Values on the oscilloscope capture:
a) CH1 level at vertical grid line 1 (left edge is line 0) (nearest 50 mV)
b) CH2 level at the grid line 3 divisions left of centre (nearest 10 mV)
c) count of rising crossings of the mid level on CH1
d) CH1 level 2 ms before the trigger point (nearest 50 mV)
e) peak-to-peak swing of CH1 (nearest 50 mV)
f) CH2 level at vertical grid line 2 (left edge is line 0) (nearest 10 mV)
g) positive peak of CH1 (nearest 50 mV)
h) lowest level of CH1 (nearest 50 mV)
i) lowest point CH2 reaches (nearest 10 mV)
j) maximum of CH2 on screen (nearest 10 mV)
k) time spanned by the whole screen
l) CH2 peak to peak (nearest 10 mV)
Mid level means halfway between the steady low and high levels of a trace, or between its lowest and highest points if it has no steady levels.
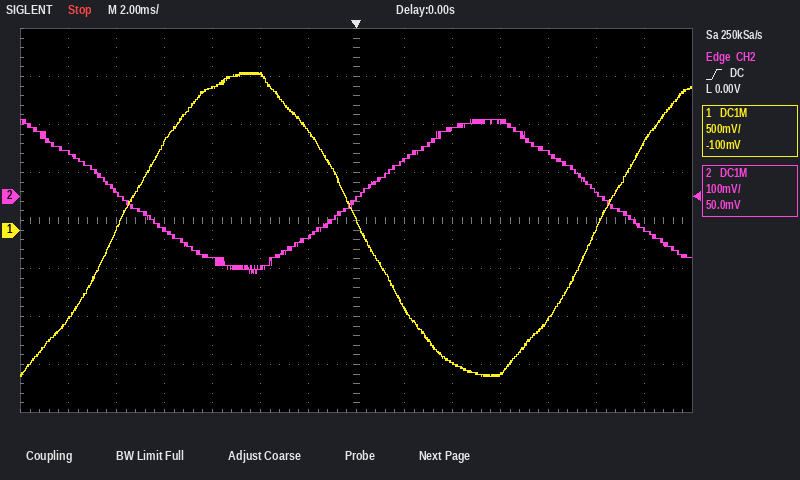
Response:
-950 mV
-130 mV
2
1.05 V
3.15 V
10 mV
1.65 V
-1.50 V
-160 mV
160 mV
28 ms
320 mV
